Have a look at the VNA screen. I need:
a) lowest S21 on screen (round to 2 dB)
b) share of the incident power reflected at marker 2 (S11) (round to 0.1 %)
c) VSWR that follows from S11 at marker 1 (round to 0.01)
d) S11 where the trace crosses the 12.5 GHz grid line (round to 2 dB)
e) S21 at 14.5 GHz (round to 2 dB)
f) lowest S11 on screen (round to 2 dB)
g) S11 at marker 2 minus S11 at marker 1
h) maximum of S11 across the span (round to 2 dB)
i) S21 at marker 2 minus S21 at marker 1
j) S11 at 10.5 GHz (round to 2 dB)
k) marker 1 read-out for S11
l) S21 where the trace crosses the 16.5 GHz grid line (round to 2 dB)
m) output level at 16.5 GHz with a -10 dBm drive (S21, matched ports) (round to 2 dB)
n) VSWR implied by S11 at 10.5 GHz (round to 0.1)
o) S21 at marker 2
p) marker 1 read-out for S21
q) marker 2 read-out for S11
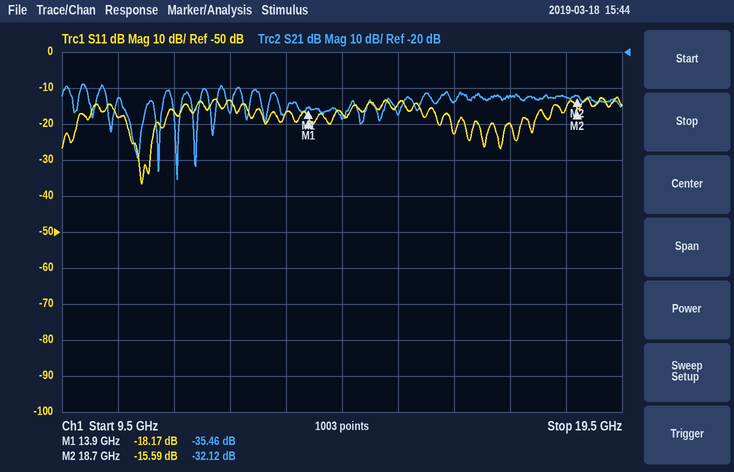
-56 dB
2.8 %
1.28
-14 dB
-38 dB
-36 dB
2.58 dB
-12 dB
3.34 dB
-18 dB
-18.17 dB
-34 dB
-44 dBm
1.3
-32.12 dB
-35.46 dB
-15.59 dB
